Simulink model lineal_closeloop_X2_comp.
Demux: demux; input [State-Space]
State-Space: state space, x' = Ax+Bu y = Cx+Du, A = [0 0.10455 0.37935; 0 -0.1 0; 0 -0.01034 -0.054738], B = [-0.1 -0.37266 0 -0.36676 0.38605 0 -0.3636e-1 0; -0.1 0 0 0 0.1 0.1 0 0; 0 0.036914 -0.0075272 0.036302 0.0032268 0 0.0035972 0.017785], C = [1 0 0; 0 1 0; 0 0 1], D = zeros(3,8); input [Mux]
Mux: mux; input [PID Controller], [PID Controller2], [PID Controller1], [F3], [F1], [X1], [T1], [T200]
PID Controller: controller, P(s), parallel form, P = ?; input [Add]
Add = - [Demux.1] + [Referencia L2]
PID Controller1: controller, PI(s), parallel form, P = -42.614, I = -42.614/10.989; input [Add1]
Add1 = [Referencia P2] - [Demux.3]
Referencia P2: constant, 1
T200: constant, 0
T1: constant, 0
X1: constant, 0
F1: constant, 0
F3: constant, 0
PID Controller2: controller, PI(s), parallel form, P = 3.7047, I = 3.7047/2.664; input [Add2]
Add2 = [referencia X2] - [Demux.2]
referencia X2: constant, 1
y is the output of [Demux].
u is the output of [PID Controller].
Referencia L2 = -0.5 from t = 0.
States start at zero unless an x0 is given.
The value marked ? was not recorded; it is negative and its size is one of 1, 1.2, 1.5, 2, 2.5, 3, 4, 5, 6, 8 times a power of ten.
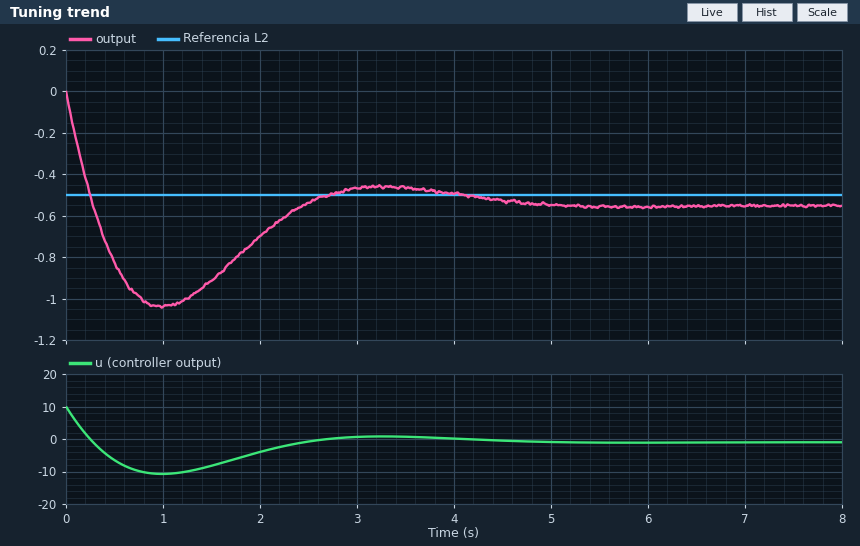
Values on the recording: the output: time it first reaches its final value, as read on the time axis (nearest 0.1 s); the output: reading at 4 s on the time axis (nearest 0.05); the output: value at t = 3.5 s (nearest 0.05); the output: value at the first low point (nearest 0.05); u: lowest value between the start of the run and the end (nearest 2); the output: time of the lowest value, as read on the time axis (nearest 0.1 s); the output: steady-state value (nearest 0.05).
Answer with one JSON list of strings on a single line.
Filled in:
["0.3 s", "-0.50", "-0.45", "-1.05", "-10", "1.0 s", "-0.55"]
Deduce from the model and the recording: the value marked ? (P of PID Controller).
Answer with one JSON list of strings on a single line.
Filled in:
["-20"]
